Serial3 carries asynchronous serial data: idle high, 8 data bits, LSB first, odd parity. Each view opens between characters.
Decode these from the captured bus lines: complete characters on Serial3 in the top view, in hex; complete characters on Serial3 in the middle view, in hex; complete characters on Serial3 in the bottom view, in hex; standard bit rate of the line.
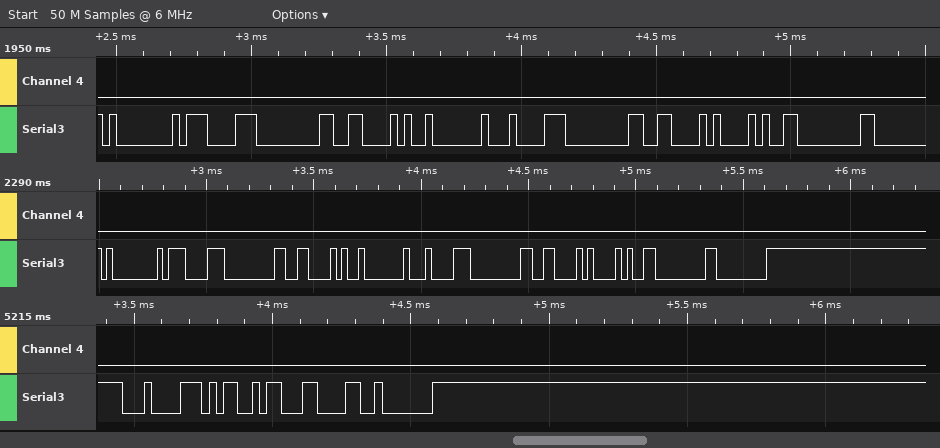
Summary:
01, 87, 00, 86, 02, 84, 00, 86, 28, 00
01, 87, 00, 86, 02, 84, 00, 86, 28, 00, 00
84, 4D, 0C, 02
38400 baud
